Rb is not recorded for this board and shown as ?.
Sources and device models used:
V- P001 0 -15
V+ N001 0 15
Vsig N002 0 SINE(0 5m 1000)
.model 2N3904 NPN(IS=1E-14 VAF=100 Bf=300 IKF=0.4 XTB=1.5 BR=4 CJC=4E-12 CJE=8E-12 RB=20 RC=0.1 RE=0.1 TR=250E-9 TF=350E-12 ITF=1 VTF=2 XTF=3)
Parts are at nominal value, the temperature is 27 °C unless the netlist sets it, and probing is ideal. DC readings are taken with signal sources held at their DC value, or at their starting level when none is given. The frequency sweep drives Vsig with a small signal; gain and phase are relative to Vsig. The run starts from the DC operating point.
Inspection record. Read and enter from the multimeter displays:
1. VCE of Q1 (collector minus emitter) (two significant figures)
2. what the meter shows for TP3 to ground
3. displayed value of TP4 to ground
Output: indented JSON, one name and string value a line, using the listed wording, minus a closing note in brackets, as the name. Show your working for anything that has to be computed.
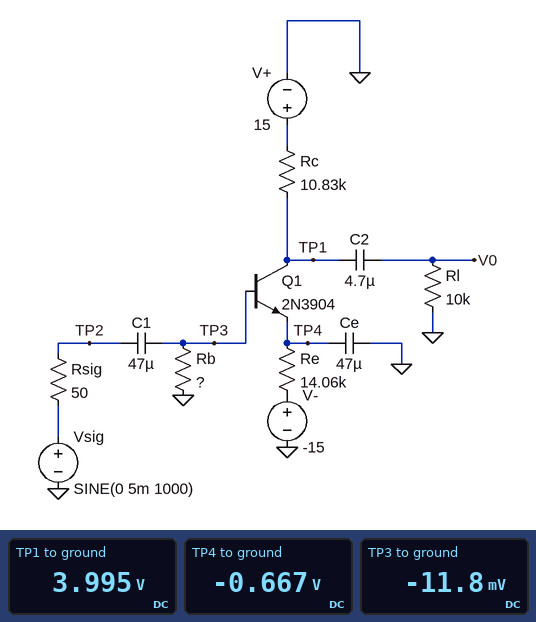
{
  "VCE of Q1 (collector minus emitter)": "3.995 V - (-667 mV) = 4.7 V",
  "what the meter shows for TP3 to ground": "-11.8 mV",
  "displayed value of TP4 to ground": "-0.667 V"
}
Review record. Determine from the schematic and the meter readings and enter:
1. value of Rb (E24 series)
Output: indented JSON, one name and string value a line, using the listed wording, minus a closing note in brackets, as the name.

{
  "value of Rb": "3.6 kΩ"
}
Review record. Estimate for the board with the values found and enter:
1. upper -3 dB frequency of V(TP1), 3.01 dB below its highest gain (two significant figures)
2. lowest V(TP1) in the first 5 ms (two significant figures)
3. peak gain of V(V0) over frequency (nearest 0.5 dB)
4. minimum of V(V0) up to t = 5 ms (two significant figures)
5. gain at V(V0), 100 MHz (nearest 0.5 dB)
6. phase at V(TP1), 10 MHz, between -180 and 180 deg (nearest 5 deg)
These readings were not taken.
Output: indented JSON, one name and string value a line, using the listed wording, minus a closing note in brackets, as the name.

{
  "upper -3 dB frequency of V(TP1), 3.01 dB below its highest gain": "3.9 MHz",
  "lowest V(TP1) in the first 5 ms": "3.0 V",
  "peak gain of V(V0) over frequency": "45.5 dB",
  "minimum of V(V0) up to t = 5 ms": "-970 mV",
  "gain at V(V0), 100 MHz": "17.0 dB",
  "phase at V(TP1), 10 MHz, between -180 and 180 deg": "110 deg"
}
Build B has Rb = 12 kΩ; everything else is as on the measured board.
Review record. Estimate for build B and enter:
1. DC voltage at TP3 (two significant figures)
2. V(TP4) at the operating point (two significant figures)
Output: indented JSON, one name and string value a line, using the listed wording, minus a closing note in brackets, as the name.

{
  "DC voltage at TP3": "-39 mV",
  "V(TP4) at the operating point": "-690 mV"
}
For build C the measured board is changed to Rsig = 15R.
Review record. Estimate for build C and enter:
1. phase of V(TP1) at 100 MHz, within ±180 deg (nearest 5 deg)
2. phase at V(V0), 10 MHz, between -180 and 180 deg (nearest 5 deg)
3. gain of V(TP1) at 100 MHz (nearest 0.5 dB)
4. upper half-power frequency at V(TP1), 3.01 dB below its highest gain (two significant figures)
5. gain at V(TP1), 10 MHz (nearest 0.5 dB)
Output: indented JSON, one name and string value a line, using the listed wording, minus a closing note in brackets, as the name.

{
  "phase of V(TP1) at 100 MHz, within ±180 deg": "80 deg",
  "phase at V(V0), 10 MHz, between -180 and 180 deg": "120 deg",
  "gain of V(TP1) at 100 MHz": "21.0 dB",
  "upper half-power frequency at V(TP1), 3.01 dB below its highest gain": "6.1 MHz",
  "gain at V(TP1), 10 MHz": "40.0 dB"
}
